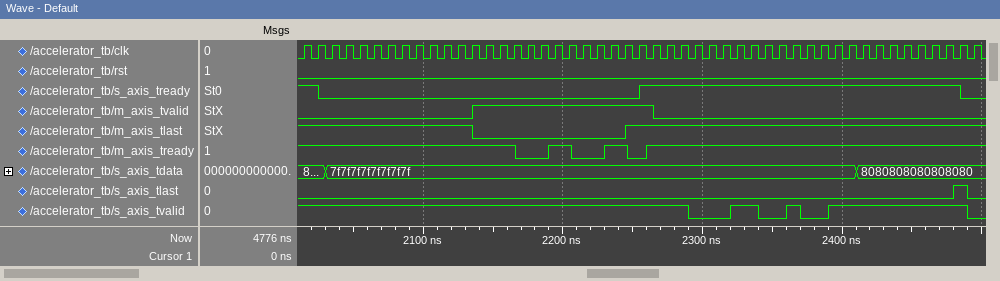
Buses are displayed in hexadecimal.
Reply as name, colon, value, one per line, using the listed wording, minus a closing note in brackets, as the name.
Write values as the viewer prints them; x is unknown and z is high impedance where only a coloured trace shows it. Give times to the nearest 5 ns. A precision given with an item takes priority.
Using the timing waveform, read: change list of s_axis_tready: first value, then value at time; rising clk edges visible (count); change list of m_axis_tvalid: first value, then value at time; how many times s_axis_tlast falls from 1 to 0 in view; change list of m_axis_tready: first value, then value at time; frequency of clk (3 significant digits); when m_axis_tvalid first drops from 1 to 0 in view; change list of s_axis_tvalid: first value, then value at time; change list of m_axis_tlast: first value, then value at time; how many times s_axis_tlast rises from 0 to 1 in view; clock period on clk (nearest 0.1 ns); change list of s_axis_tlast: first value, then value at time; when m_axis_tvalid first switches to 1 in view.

change list of s_axis_tready: first value, then value at time: 1, 0 at 2025 ns, 1 at 2255 ns, 0 at 2485 ns
rising clk edges visible: 49
change list of m_axis_tvalid: first value, then value at time: 0, 1 at 2135 ns, 0 at 2265 ns
how many times s_axis_tlast falls from 1 to 0 in view: 1
change list of m_axis_tready: first value, then value at time: 1, 0 at 2165 ns, 1 at 2190 ns, 0 at 2205 ns, 1 at 2230 ns, 0 at 2245 ns, 1 at 2260 ns
frequency of clk: 100 MHz
when m_axis_tvalid first drops from 1 to 0 in view: 2265 ns
change list of s_axis_tvalid: first value, then value at time: 1, 0 at 2290 ns, 1 at 2320 ns, 0 at 2340 ns, 1 at 2360 ns, 0 at 2370 ns, 1 at 2390 ns, 0 at 2490 ns
change list of m_axis_tlast: first value, then value at time: 1, 0 at 2135 ns, 1 at 2245 ns
how many times s_axis_tlast rises from 0 to 1 in view: 1
clock period on clk: 10 ns
change list of s_axis_tlast: first value, then value at time: 0, 1 at 2480 ns, 0 at 2490 ns
when m_axis_tvalid first switches to 1 in view: 2135 ns
